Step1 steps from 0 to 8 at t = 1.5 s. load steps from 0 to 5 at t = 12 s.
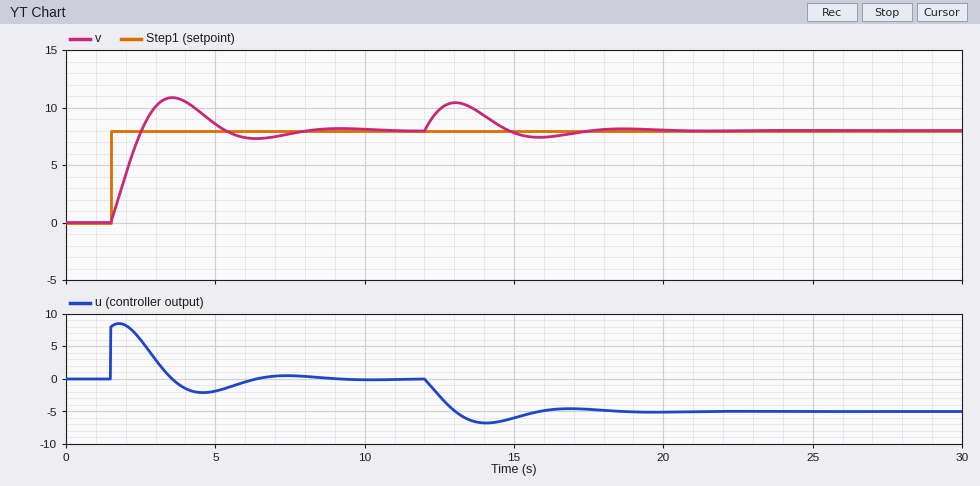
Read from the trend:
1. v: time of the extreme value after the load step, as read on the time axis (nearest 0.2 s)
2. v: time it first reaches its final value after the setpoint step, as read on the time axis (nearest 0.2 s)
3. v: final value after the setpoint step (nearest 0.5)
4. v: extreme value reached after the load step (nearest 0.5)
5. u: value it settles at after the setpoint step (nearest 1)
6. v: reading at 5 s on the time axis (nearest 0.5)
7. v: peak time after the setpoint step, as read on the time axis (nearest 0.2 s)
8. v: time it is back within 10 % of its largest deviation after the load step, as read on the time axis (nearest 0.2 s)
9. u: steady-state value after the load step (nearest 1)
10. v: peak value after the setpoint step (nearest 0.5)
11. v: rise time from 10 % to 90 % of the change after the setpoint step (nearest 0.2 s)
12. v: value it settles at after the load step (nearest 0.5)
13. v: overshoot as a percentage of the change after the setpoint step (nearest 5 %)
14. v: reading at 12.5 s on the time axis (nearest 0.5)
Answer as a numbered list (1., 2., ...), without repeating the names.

1. 13.0 s
2. 2.6 s
3. 8.0
4. 10.5
5. 0
6. 8.5
7. 3.6 s
8. 17.0 s
9. -5
10. 11.0
11. 0.8 s
12. 8.0
13. 35 %
14. 10.0
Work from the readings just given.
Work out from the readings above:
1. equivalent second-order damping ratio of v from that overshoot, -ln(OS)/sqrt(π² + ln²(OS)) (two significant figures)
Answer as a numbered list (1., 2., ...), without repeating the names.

1. 0.32
